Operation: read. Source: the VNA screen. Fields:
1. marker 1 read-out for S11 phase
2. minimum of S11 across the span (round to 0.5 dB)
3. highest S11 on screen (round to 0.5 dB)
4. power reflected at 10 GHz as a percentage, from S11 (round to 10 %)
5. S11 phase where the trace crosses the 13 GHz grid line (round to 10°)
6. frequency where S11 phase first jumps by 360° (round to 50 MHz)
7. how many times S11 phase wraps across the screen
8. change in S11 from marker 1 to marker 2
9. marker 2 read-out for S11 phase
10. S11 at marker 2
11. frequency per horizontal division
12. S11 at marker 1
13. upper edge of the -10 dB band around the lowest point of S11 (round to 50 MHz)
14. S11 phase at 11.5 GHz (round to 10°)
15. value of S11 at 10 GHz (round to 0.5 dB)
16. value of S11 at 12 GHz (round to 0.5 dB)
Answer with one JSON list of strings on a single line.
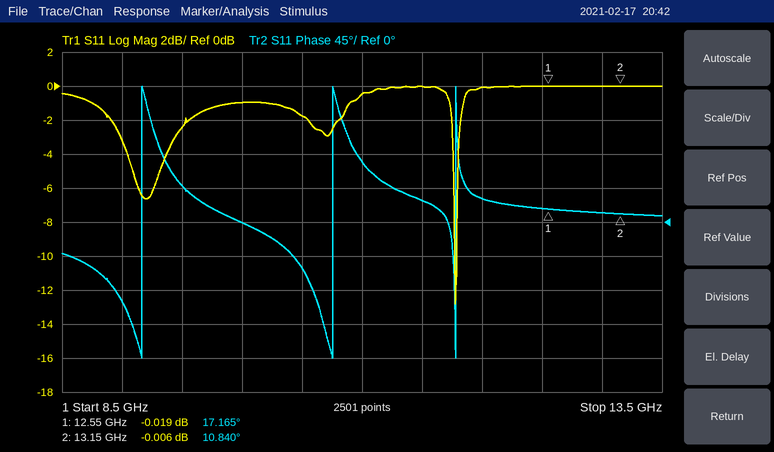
["17.165°", "-13.0 dB", "0.0 dB", "80 %", "10°", "9.15 GHz", "3", "0.013 dB", "10.840°", "-0.006 dB", "500 MHz", "-0.019 dB", "11.80 GHz", "30°", "-1.0 dB", "0.0 dB"]
